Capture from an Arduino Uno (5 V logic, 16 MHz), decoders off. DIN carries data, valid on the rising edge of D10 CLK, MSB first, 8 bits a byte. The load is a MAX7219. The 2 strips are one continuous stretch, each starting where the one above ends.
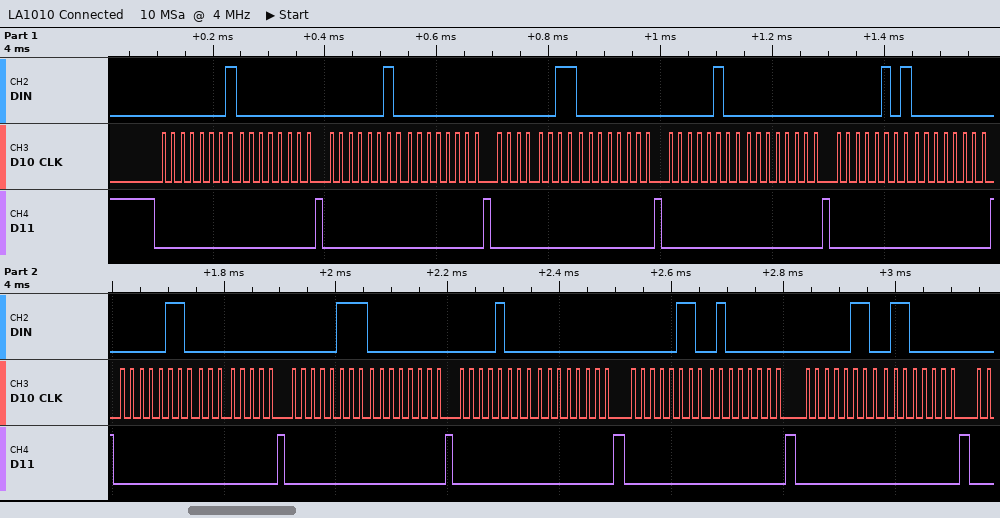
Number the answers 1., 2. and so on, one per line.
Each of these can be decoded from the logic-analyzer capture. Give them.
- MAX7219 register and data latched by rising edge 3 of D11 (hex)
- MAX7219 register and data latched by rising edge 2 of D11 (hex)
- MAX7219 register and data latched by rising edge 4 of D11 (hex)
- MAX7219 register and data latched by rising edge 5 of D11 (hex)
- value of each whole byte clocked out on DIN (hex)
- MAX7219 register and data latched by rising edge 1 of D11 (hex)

1. register 0x3, data 0x00
2. register 0x2, data 0x00
3. register 0x4, data 0x00
4. register 0x5, data 0x00
5. 0x01 0x00 0x02 0x00 0x03 0x00 0x04 0x00 0x05 0x00 0x06 0x00 0x07 0x00 0x08 0x00 0x06 0x40 0x06 0x60
6. register 0x1, data 0x00
